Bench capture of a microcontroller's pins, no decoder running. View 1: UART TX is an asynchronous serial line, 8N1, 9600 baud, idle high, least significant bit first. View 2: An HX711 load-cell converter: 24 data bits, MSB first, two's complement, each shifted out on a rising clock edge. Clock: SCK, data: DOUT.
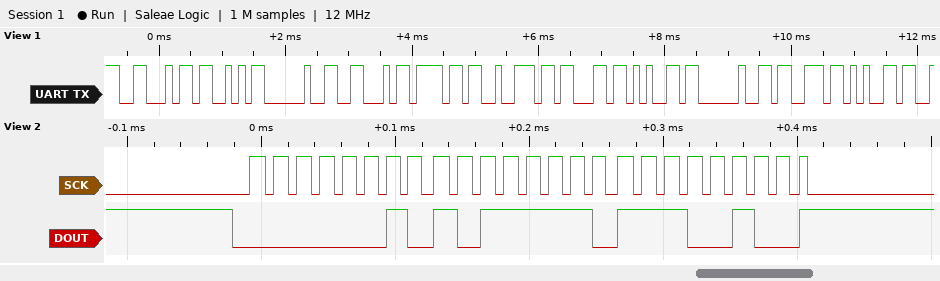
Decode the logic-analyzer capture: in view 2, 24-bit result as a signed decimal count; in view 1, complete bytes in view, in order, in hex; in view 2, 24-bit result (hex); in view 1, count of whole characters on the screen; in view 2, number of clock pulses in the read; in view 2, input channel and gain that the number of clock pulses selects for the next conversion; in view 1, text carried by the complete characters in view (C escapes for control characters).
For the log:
179940
46 53 20 46 6F 72 63 65 20 73 65
0x02BEE4
11
25
channel A, gain 128
"FS Force se"
